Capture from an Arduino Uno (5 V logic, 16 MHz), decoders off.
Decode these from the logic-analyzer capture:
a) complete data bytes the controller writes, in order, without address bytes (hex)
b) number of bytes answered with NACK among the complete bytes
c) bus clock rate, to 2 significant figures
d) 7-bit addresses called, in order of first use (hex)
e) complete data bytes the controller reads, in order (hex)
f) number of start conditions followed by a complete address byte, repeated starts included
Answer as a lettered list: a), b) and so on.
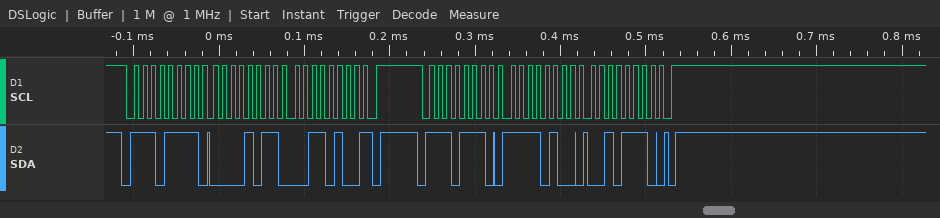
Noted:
a) F4 2E
b) 1
c) 100 kHz
d) 0x77
e) 0B 34
f) 2
